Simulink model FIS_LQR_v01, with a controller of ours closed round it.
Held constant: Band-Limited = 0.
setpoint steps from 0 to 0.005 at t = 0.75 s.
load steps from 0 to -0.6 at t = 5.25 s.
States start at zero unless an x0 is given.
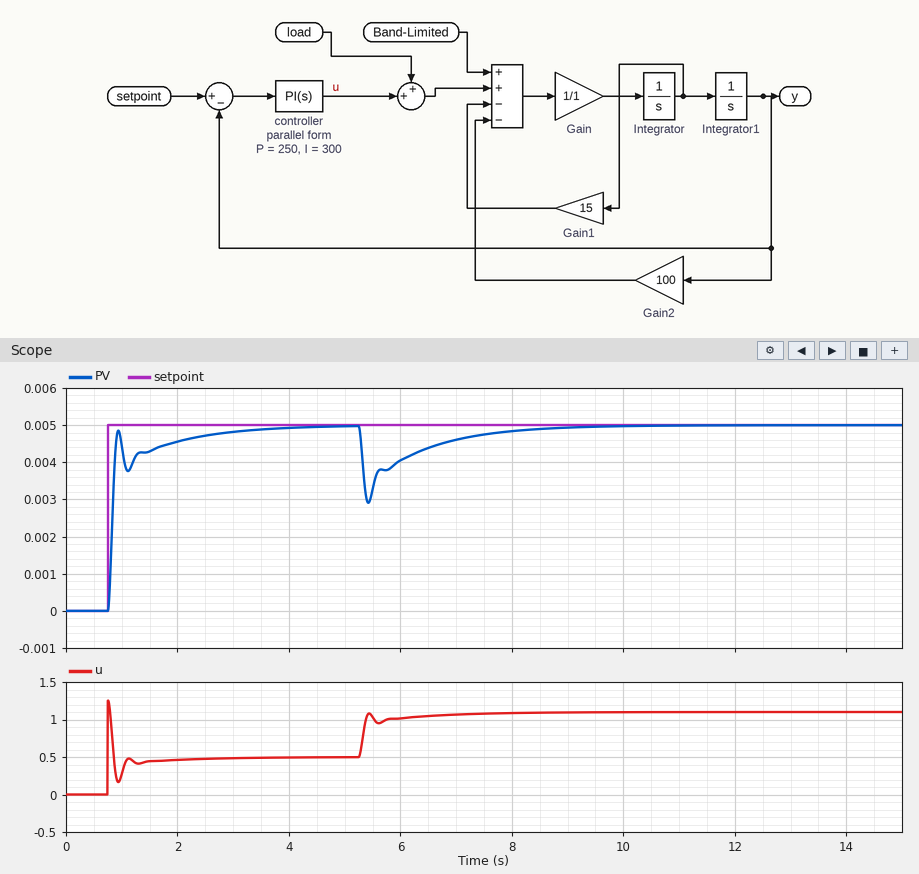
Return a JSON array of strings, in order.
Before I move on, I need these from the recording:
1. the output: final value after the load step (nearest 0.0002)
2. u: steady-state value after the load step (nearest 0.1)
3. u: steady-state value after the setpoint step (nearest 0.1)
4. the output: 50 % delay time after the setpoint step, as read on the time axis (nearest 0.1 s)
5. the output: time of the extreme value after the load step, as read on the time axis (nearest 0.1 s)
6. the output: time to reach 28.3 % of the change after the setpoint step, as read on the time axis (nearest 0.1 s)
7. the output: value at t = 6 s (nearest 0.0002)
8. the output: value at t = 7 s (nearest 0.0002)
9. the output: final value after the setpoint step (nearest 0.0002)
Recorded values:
["0.0050", "1.1", "0.5", "0.8 s", "5.4 s", "0.8 s", "0.0040", "0.0046", "0.0050"]
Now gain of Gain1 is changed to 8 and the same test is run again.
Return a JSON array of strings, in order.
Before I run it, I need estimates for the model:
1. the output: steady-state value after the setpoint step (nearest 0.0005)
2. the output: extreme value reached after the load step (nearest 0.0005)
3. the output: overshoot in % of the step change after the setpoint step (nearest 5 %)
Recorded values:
["0.0050", "0.0025", "15 %"]
